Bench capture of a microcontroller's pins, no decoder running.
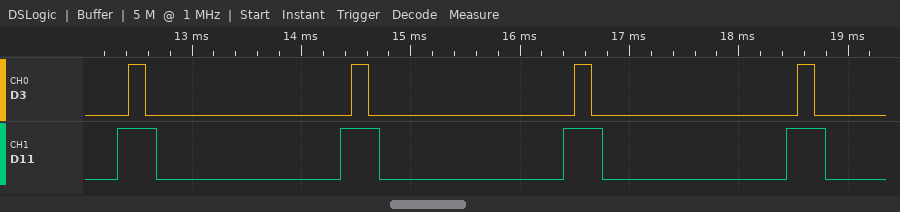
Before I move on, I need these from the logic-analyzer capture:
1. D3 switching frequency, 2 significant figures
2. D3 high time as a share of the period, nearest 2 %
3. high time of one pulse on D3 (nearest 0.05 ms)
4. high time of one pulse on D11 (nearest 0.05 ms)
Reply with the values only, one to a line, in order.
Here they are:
490 Hz
8 %
0.15 ms
0.35 ms
